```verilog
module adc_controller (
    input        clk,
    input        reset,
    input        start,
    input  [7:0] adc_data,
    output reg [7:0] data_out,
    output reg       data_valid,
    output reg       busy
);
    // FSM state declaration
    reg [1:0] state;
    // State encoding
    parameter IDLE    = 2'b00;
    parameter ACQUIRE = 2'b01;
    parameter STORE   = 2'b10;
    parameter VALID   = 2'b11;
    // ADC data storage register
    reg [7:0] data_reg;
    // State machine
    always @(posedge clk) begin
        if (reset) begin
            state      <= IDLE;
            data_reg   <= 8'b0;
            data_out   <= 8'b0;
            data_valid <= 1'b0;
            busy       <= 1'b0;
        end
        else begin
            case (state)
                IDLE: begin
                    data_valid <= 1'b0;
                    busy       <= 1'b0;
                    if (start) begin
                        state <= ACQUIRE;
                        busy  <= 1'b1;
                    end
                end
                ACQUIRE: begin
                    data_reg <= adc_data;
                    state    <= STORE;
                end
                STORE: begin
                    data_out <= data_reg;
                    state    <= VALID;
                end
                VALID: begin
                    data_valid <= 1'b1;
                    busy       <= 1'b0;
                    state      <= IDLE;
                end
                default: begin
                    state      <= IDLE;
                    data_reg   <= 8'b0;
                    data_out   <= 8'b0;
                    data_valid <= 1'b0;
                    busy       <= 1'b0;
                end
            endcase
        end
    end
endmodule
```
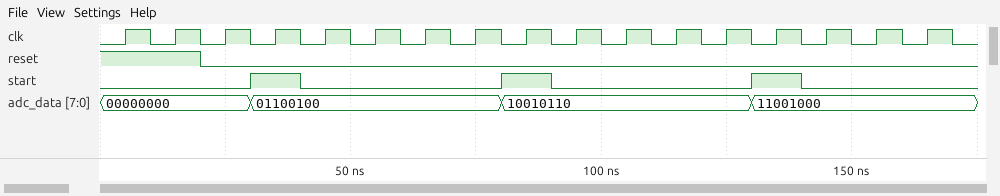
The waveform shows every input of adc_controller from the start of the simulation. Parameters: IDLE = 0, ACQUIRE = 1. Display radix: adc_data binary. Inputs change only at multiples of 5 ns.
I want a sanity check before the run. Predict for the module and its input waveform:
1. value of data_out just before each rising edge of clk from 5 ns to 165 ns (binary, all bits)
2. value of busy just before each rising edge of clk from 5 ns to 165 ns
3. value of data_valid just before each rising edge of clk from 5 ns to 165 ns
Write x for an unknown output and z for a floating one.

x, 00000000, 00000000, 00000000, 00000000, 00000000, 01100100, 01100100, 01100100, 01100100, 01100100, 10010110, 10010110, 10010110, 10010110, 10010110, 11001000
x 0 0 0 1 1 1 0 0 1 1 1 0 0 1 1 1
x 0 0 0 0 0 0 1 0 0 0 0 1 0 0 0 0
